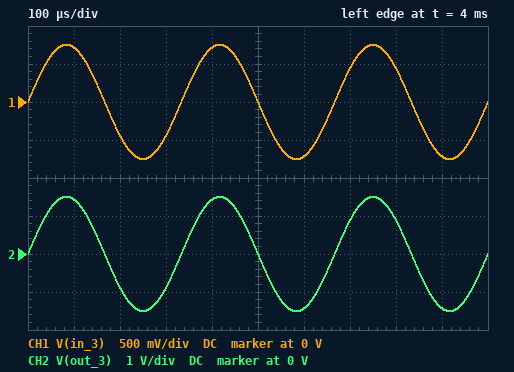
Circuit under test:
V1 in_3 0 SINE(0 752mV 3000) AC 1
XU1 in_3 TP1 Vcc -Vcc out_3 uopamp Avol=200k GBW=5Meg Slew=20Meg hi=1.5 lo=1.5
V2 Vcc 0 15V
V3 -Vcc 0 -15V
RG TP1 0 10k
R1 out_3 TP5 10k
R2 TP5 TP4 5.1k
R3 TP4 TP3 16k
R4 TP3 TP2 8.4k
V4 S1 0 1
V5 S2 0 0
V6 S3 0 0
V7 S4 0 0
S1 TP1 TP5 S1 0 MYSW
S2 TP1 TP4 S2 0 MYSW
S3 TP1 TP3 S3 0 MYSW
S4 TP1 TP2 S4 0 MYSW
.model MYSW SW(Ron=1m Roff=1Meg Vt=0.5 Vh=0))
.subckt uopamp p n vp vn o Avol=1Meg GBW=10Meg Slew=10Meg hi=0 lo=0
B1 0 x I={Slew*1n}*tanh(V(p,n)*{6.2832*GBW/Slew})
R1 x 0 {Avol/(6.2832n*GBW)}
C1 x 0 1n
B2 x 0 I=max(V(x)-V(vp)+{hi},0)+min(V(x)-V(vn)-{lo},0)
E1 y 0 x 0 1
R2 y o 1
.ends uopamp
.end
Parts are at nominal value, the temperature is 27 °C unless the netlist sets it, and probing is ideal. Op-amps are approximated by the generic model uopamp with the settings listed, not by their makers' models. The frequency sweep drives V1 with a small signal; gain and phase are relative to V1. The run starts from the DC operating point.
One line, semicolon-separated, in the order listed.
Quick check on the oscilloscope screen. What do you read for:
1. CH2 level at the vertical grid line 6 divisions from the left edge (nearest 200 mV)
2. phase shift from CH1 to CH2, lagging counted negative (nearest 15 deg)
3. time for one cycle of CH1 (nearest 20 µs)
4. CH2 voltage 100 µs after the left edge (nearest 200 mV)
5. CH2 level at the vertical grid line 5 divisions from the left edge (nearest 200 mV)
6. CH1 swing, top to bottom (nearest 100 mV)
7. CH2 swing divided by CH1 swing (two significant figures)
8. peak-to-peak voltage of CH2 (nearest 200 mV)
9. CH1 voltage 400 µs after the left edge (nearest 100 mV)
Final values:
-1.4 V; 0 deg; 340 µs; 1.4 V; 0 V; 1.5 V; 2.0; 3.0 V; 700 mV
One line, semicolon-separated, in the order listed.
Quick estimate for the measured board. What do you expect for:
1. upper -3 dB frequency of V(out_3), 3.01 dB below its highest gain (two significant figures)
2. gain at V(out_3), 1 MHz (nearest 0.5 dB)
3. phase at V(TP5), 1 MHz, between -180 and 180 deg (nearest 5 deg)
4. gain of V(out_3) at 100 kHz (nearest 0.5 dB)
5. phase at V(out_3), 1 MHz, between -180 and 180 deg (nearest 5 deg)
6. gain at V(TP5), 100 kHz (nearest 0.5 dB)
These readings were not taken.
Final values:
180 kHz; 14.0 dB; -80 deg; 27.5 dB; -80 deg; 27.5 dB
